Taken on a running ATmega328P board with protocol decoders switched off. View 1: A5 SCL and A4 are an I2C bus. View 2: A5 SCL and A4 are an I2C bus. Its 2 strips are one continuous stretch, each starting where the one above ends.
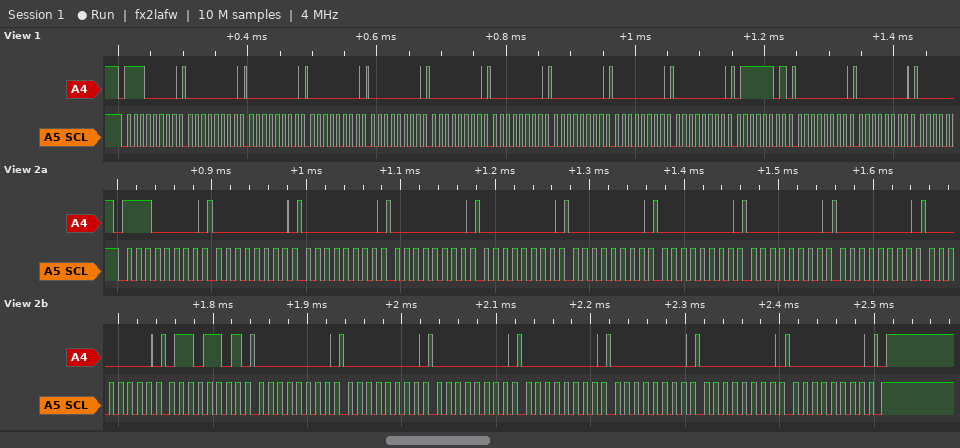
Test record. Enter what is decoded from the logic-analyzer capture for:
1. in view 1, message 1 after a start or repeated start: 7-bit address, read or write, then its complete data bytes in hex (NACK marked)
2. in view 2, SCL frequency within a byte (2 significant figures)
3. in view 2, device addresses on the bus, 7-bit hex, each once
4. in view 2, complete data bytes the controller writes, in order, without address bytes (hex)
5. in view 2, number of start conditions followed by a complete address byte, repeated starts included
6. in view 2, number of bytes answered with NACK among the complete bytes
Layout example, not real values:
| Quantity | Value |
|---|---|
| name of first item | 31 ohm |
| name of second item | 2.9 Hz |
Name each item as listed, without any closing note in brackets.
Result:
| Quantity | Value |
|---|---|
| in view 1, message 1 after a start or repeated start: 7-bit address, read or write, then its complete data bytes in hex | 0x70 write: 00 00 00 00 00 00 00 00 00 7D 00 00 |
| in view 2, SCL frequency within a byte | 100 kHz |
| in view 2, device addresses on the bus, 7-bit hex, each once | 0x70 |
| in view 2, complete data bytes the controller writes, in order, without address bytes | 00 00 00 00 00 00 00 00 00 6D 00 00 00 00 00 00 00 |
| in view 2, number of start conditions followed by a complete address byte, repeated starts included | 1 |
| in view 2, number of bytes answered with NACK among the complete bytes | 0 |
